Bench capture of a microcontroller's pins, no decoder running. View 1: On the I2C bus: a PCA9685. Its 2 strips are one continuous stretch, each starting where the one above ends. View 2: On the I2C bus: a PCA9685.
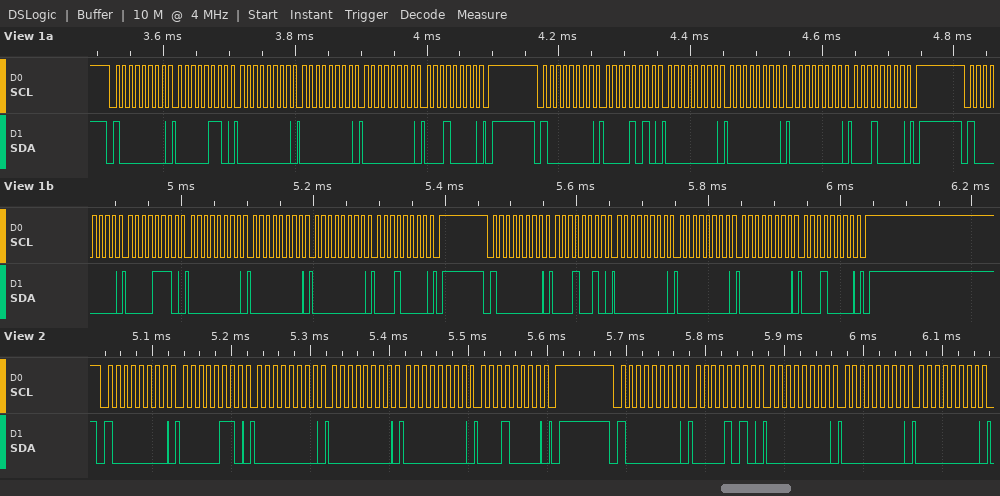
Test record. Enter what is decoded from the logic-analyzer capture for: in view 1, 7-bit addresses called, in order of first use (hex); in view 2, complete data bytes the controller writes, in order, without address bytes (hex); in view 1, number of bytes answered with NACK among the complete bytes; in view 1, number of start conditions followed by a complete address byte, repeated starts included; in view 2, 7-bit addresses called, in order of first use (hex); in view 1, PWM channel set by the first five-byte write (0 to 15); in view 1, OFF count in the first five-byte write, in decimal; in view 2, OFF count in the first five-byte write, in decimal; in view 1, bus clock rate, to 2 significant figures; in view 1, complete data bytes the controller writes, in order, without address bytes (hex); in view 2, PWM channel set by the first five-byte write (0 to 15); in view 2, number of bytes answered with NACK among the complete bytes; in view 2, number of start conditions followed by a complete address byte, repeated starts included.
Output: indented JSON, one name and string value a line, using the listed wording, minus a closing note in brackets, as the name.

{
  "in view 1, 7-bit addresses called, in order of first use": "0x40",
  "in view 2, complete data bytes the controller writes, in order, without address bytes": "06 00 00 00 10 0A 00 00 00",
  "in view 1, number of bytes answered with NACK among the complete bytes": "0",
  "in view 1, number of start conditions followed by a complete address byte, repeated starts included": "4",
  "in view 2, 7-bit addresses called, in order of first use": "0x40",
  "in view 1, PWM channel set by the first five-byte write": "0",
  "in view 1, OFF count in the first five-byte write, in decimal": "4096",
  "in view 2, OFF count in the first five-byte write, in decimal": "4096",
  "in view 1, bus clock rate, to 2 significant figures": "100 kHz",
  "in view 1, complete data bytes the controller writes, in order, without address bytes": "06 00 00 00 10 0A 00 00 00 10 0E 00 00 00 10 12 00 00 00 10",
  "in view 2, PWM channel set by the first five-byte write": "0",
  "in view 2, number of bytes answered with NACK among the complete bytes": "0",
  "in view 2, number of start conditions followed by a complete address byte, repeated starts included": "2"
}
